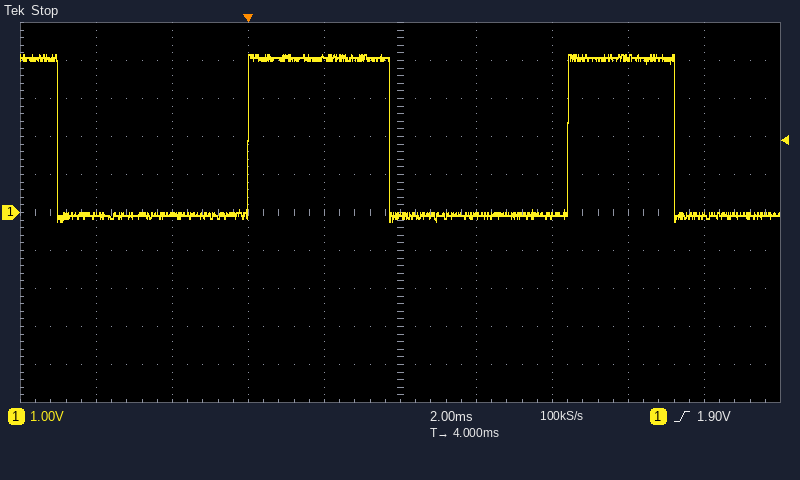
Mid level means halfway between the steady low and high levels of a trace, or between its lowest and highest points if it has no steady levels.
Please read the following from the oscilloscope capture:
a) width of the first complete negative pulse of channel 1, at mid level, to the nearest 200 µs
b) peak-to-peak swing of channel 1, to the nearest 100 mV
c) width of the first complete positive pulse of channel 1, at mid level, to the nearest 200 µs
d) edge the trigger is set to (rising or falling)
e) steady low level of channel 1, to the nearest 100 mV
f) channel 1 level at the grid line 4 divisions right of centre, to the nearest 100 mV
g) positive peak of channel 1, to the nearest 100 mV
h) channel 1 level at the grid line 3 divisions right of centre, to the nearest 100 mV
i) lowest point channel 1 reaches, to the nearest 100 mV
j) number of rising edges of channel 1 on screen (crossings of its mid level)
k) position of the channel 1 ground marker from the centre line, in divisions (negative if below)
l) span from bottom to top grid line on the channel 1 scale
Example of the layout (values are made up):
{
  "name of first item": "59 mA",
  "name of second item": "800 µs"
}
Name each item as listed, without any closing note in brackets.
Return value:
{
  "width of the first complete negative pulse of channel 1, at mid level, to the nearest 200 µs": "5.0 ms",
  "peak-to-peak swing of channel 1, to the nearest 100 mV": "4.4 V",
  "width of the first complete positive pulse of channel 1, at mid level, to the nearest 200 µs": "3.8 ms",
  "edge the trigger is set to": "rising",
  "steady low level of channel 1, to the nearest 100 mV": "-100 mV",
  "channel 1 level at the grid line 4 divisions right of centre, to the nearest 100 mV": "-100 mV",
  "positive peak of channel 1, to the nearest 100 mV": "4.2 V",
  "channel 1 level at the grid line 3 divisions right of centre, to the nearest 100 mV": "4.1 V",
  "lowest point channel 1 reaches, to the nearest 100 mV": "-200 mV",
  "number of rising edges of channel 1 on screen": "2",
  "position of the channel 1 ground marker from the centre line, in divisions": "0.0 div",
  "span from bottom to top grid line on the channel 1 scale": "10 V"
}
